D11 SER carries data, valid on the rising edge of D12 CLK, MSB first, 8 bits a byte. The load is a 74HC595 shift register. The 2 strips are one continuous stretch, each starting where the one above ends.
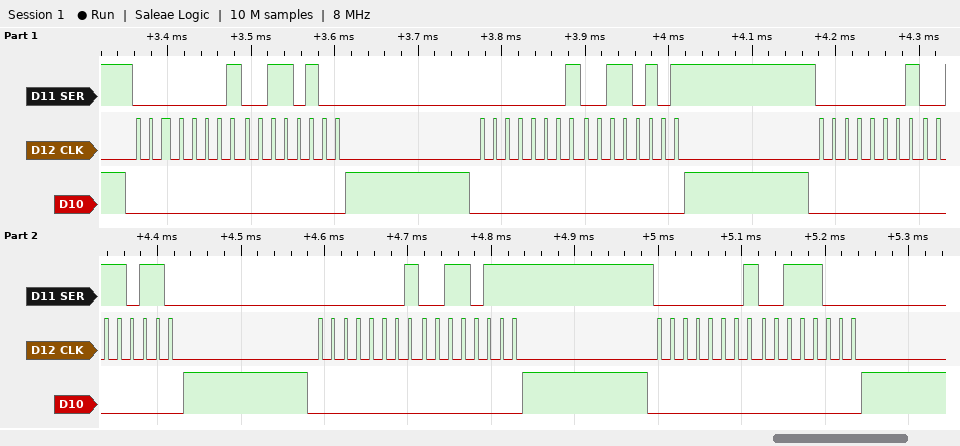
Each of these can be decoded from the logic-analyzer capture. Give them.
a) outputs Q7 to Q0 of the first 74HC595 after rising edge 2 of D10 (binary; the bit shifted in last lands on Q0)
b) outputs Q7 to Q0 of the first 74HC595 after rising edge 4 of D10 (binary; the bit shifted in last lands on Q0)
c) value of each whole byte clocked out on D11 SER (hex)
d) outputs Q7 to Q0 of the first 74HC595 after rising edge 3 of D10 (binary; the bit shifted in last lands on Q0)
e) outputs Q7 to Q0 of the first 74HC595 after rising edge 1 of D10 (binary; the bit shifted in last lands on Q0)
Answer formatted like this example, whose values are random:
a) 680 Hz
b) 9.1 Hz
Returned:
a) 00110101
b) 00110111
c) 01 34 01 35 01 36 01 37 01 38
d) 00110110
e) 00110100
